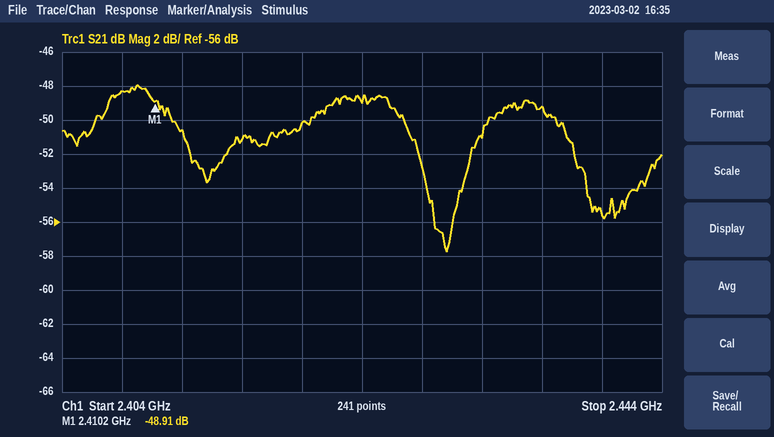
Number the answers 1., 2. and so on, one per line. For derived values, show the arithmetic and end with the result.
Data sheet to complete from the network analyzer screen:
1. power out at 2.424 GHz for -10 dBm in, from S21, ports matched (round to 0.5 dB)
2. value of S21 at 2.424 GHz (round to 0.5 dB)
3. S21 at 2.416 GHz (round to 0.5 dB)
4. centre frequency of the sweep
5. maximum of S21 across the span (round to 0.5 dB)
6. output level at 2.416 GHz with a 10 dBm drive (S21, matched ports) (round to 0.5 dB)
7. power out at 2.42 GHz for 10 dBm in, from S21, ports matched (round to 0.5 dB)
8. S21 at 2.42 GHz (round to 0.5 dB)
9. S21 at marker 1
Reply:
1. -10 dBm + (-49.0 dB) = -59.0 dBm
2. -49.0 dB
3. -51.0 dB
4. 2.424 GHz
5. -48.0 dB
6. 10 dBm + (-51.0 dB) = -41.0 dBm
7. 10 dBm + (-50.0 dB) = -40.0 dBm
8. -50.0 dB
9. -48.91 dB
